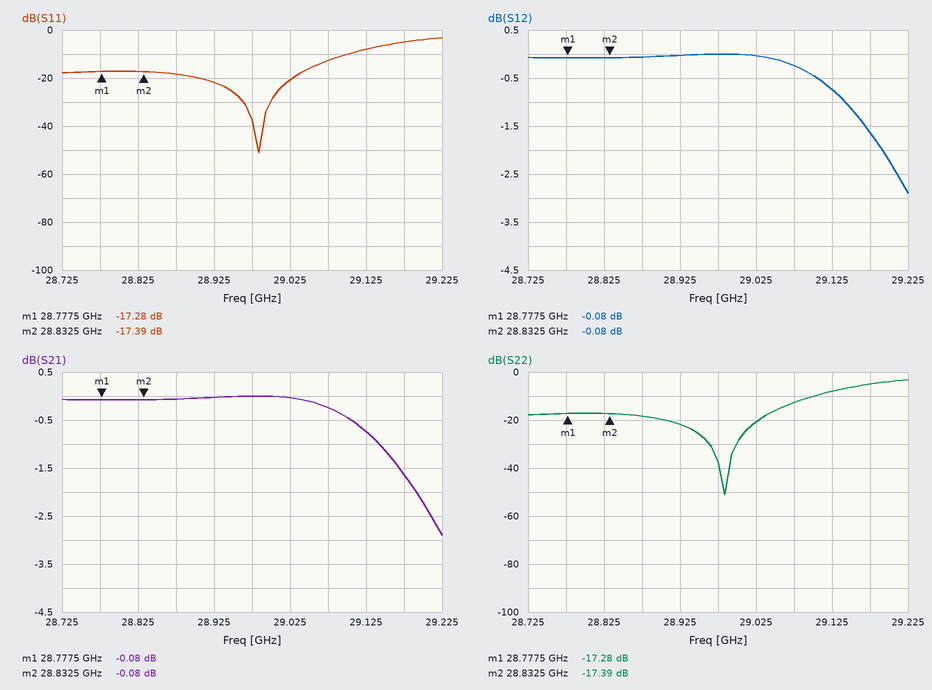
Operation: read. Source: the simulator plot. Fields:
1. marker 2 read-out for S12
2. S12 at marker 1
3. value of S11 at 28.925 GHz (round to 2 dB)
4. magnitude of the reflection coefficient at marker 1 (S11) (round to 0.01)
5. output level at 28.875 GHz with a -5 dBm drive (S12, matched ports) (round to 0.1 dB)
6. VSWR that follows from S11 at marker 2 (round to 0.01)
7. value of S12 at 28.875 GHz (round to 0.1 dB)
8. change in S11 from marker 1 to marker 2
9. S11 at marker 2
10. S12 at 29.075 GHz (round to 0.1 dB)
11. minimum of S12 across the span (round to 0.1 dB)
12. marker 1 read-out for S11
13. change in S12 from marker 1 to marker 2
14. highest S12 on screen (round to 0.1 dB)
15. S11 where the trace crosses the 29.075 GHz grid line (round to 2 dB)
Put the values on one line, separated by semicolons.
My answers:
-0.08 dB; -0.08 dB; -22 dB; 0.14; -5.1 dBm; 1.31; -0.1 dB; -0.11 dB; -17.39 dB; -0.2 dB; -2.9 dB; -17.28 dB; 0.00 dB; 0.0 dB; -12 dB
